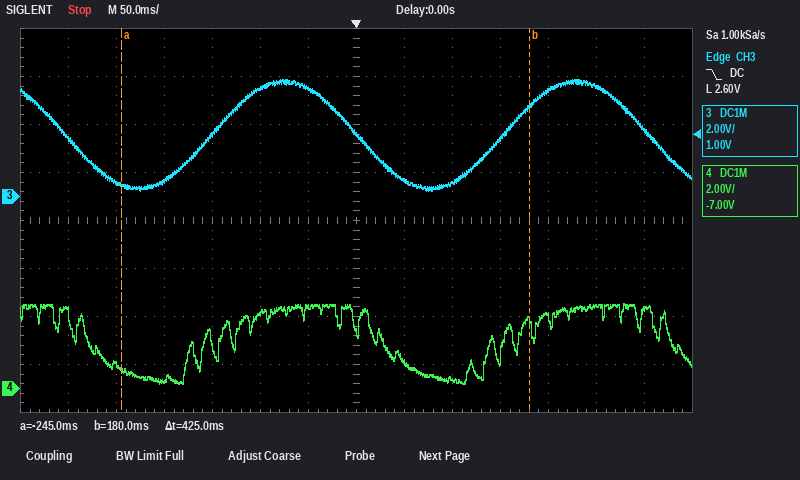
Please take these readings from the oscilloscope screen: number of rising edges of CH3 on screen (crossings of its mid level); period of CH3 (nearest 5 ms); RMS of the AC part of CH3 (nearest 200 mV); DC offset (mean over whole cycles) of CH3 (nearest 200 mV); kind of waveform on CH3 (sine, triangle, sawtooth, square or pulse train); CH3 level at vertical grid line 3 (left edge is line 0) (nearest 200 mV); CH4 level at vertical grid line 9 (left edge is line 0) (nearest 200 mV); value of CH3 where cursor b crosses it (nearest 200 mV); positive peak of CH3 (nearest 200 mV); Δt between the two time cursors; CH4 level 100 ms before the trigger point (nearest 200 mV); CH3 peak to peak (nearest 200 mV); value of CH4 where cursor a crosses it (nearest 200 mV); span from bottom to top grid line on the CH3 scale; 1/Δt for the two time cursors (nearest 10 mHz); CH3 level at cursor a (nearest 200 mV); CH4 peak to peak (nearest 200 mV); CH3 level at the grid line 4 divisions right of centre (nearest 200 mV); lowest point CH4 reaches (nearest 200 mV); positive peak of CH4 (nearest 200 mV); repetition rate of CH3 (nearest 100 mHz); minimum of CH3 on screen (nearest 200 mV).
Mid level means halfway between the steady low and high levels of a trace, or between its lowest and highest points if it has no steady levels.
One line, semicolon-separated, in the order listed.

2; 305 ms; 1.6 V; 2.6 V; sine; 600 mV; 400 mV; 3.8 V; 4.8 V; 425 ms; 3.2 V; 4.6 V; 800 mV; 16 V; 2.35 Hz; 400 mV; 3.4 V; 4.4 V; 200 mV; 3.6 V; 3.3 Hz; 200 mV
